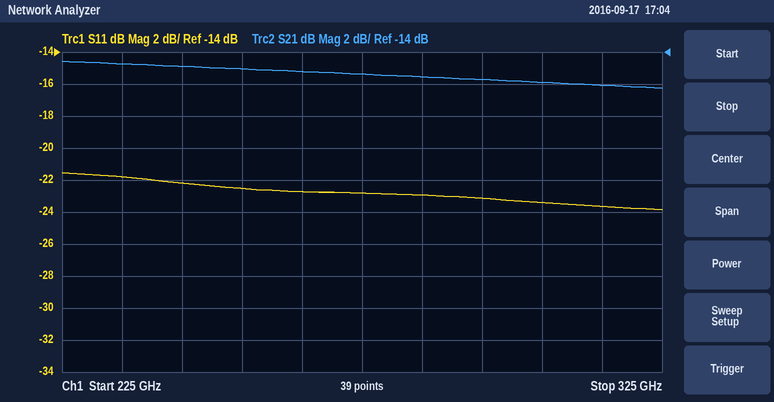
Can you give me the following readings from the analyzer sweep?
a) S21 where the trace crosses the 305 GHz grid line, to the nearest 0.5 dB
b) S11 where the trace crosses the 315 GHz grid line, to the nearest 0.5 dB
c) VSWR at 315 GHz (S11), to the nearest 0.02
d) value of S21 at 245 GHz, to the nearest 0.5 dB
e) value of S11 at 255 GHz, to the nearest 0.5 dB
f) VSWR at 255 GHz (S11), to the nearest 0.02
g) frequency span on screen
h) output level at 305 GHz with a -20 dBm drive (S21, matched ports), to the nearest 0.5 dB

-16.0 dB
-23.5 dB
1.14
-15.0 dB
-22.5 dB
1.16
100 GHz
-36.0 dBm
